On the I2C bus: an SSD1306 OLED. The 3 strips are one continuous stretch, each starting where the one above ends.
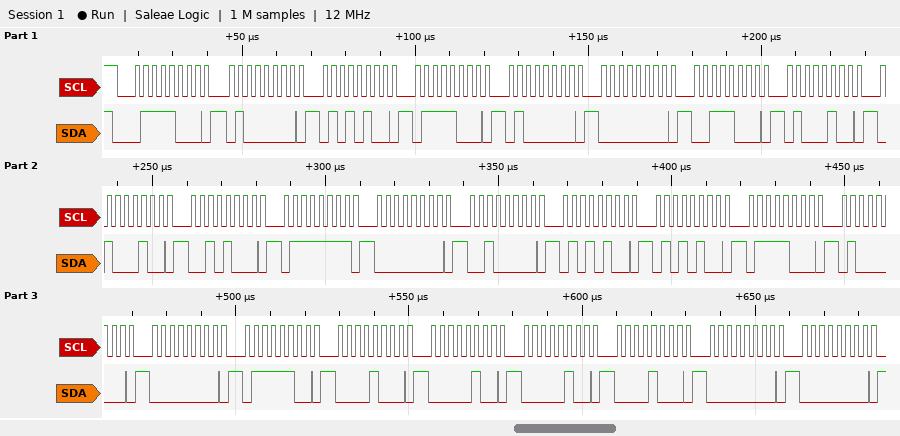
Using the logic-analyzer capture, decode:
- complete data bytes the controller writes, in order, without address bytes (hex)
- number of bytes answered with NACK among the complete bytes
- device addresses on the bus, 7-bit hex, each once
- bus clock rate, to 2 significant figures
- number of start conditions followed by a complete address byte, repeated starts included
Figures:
40 54 78 40 00 38 44 44 28 7F 00 20 54 54 78 40 00 7C 08 04 04 08 00 00
0
0x3C
400 kHz
1
